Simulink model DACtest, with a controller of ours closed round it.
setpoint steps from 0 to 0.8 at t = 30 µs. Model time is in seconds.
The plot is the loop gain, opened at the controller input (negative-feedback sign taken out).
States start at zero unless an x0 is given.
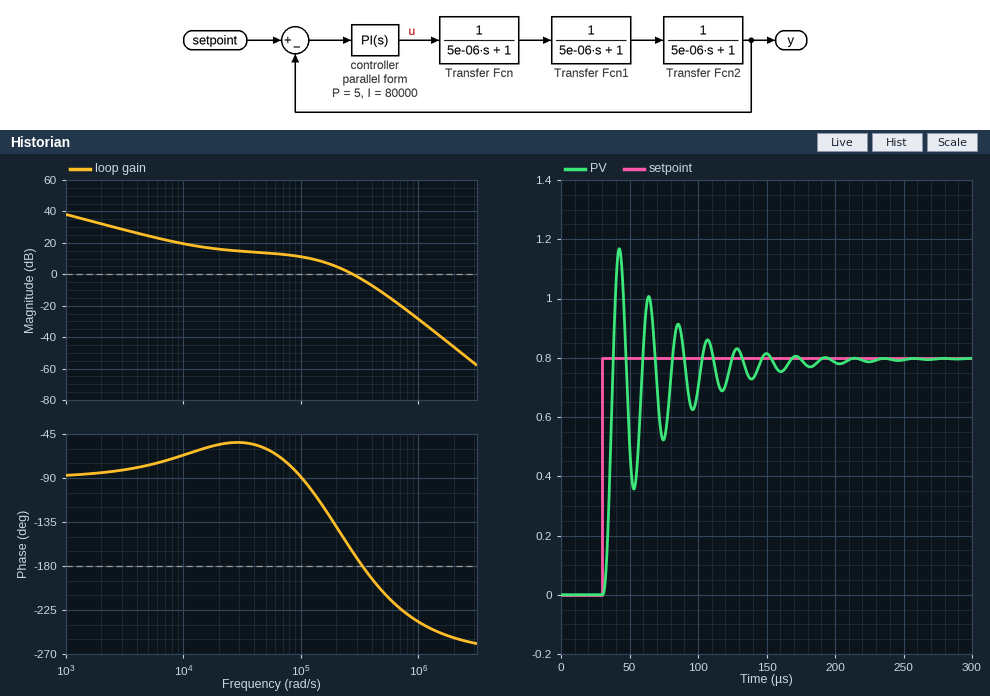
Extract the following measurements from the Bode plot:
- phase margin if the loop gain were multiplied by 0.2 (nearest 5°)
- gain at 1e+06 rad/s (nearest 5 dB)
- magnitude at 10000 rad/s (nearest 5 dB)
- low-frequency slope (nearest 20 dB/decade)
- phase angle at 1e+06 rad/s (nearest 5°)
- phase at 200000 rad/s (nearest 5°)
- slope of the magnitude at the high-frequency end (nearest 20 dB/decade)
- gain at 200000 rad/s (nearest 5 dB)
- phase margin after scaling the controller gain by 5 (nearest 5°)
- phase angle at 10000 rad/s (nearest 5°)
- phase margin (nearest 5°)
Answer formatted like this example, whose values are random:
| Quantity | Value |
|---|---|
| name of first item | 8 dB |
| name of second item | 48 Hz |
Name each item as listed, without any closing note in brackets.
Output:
| Quantity | Value |
|---|---|
| phase margin if the loop gain were multiplied by 0.2 | 125° |
| gain at 1e+06 rad/s | -30 dB |
| magnitude at 10000 rad/s | 20 dB |
| low-frequency slope | -20 dB/decade |
| phase angle at 1e+06 rad/s | -235° |
| phase at 200000 rad/s | -140° |
| slope of the magnitude at the high-frequency end | -60 dB/decade |
| gain at 200000 rad/s | 5 dB |
| phase margin after scaling the controller gain by 5 | -30° |
| phase angle at 10000 rad/s | -65° |
| phase margin | 15° |
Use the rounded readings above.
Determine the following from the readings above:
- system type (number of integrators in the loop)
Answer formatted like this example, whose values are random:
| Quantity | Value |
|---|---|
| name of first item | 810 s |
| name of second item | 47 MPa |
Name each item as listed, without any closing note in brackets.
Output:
| Quantity | Value |
|---|---|
| system type | 1 |
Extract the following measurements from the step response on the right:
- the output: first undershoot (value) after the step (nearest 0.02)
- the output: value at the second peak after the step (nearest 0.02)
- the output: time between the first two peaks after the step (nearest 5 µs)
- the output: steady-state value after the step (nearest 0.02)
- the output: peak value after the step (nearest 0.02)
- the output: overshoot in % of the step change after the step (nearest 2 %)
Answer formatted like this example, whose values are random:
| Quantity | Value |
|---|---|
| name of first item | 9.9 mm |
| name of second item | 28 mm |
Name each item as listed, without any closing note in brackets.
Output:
| Quantity | Value |
|---|---|
| the output: first undershoot (value) after the step | 0.36 |
| the output: value at the second peak after the step | 1.00 |
| the output: time between the first two peaks after the step | 20 µs |
| the output: steady-state value after the step | 0.80 |
| the output: peak value after the step | 1.16 |
| the output: overshoot in % of the step change after the step | 46 % |
